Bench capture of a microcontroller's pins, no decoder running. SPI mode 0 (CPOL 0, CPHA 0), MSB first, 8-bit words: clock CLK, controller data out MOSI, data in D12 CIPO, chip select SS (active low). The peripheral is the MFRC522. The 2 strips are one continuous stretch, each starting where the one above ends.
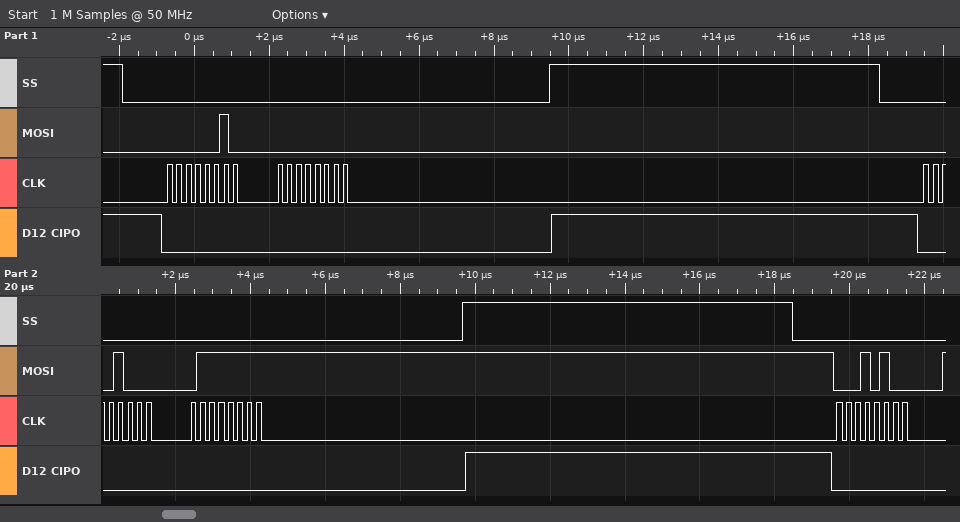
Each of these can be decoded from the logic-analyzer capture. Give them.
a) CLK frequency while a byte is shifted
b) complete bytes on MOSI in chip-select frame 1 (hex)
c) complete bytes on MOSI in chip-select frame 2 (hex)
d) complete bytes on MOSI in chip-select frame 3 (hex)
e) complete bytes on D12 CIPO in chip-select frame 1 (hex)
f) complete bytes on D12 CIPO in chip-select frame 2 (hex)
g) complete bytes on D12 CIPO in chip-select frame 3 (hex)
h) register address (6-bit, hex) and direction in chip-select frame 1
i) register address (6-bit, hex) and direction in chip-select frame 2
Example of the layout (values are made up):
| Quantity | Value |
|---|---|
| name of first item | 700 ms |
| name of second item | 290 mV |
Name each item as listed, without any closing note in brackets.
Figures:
| Quantity | Value |
|---|---|
| CLK frequency while a byte is shifted | 4 MHz |
| complete bytes on MOSI in chip-select frame 1 | 02 00 |
| complete bytes on MOSI in chip-select frame 2 | 08 7F |
| complete bytes on MOSI in chip-select frame 3 | 14 |
| complete bytes on D12 CIPO in chip-select frame 1 | 00 00 |
| complete bytes on D12 CIPO in chip-select frame 2 | 00 00 |
| complete bytes on D12 CIPO in chip-select frame 3 | 00 |
| register address (6-bit, hex) and direction in chip-select frame 1 | 0x01 write |
| register address (6-bit, hex) and direction in chip-select frame 2 | 0x04 write |
